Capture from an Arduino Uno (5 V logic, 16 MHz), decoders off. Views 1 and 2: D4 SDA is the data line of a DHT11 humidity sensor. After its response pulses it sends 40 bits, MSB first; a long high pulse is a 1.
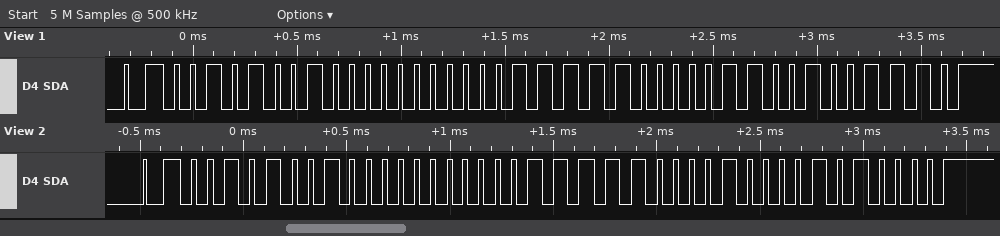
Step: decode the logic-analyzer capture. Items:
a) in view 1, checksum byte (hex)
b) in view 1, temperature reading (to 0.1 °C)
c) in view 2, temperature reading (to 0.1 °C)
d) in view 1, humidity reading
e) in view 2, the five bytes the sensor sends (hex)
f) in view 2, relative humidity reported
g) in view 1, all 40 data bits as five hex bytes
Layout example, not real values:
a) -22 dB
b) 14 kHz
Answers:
a) 0x4E
b) 31.6 °C
c) 31.8 °C
d) 41 %
e) 29 00 1F 08 50
f) 41 %
g) 29 00 1F 06 4E
